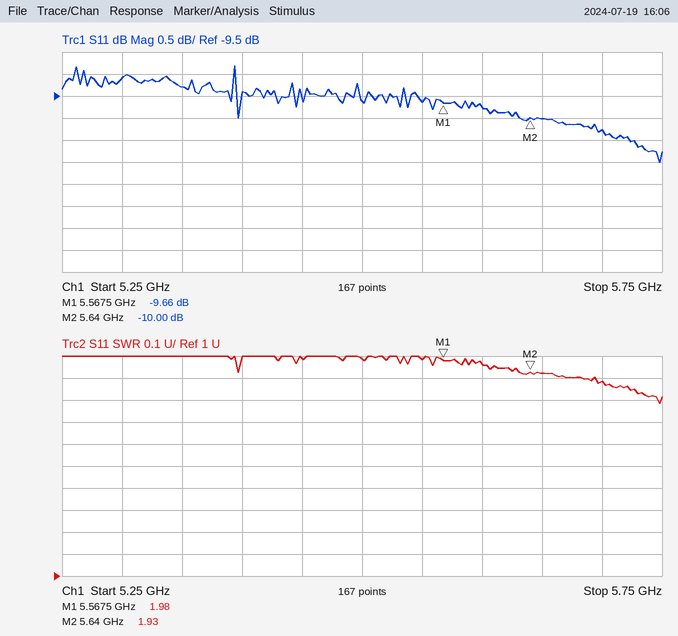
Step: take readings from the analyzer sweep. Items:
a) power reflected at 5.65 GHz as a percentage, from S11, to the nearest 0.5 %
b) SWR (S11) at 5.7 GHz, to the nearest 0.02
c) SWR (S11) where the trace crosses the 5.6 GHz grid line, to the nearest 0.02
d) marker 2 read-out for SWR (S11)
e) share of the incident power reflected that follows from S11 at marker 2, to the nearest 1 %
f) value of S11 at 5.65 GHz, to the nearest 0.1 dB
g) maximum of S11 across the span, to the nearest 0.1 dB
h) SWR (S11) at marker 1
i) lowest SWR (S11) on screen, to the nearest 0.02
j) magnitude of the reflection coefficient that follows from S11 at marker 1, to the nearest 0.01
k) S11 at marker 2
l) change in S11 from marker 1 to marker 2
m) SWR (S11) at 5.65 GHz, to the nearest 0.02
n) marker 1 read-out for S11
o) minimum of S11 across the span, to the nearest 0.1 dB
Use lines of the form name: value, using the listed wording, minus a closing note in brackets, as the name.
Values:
power reflected at 5.65 GHz as a percentage, from S11, to the nearest 0.5 %: 10.0 %
SWR (S11) at 5.7 GHz, to the nearest 0.02: 1.88
SWR (S11) where the trace crosses the 5.6 GHz grid line, to the nearest 0.02: 1.96
marker 2 read-out for SWR: 1.93
share of the incident power reflected that follows from S11 at marker 2, to the nearest 1 %: 10 %
value of S11 at 5.65 GHz, to the nearest 0.1 dB: -10.0 dB
maximum of S11 across the span, to the nearest 0.1 dB: -8.8 dB
SWR (S11) at marker 1: 1.98
lowest SWR (S11) on screen, to the nearest 0.02: 1.78
magnitude of the reflection coefficient that follows from S11 at marker 1, to the nearest 0.01: 0.33
S11 at marker 2: -10.00 dB
change in S11 from marker 1 to marker 2: -0.34 dB
SWR (S11) at 5.65 GHz, to the nearest 0.02: 1.92
marker 1 read-out for S11: -9.66 dB
minimum of S11 across the span, to the nearest 0.1 dB: -11.0 dB
